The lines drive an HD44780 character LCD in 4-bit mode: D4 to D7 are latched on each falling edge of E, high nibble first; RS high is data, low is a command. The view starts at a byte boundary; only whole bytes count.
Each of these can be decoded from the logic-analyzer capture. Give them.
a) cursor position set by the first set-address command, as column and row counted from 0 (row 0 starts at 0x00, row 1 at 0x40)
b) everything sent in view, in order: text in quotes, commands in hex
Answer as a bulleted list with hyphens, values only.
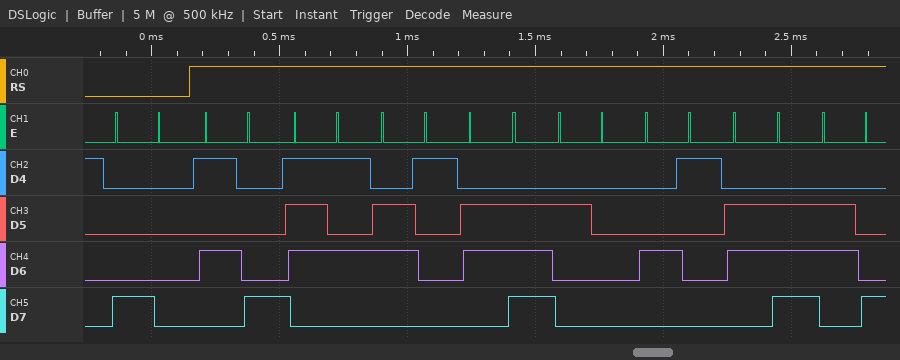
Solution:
- column 0, row 0
- 0x80 "Xuan Anh"
